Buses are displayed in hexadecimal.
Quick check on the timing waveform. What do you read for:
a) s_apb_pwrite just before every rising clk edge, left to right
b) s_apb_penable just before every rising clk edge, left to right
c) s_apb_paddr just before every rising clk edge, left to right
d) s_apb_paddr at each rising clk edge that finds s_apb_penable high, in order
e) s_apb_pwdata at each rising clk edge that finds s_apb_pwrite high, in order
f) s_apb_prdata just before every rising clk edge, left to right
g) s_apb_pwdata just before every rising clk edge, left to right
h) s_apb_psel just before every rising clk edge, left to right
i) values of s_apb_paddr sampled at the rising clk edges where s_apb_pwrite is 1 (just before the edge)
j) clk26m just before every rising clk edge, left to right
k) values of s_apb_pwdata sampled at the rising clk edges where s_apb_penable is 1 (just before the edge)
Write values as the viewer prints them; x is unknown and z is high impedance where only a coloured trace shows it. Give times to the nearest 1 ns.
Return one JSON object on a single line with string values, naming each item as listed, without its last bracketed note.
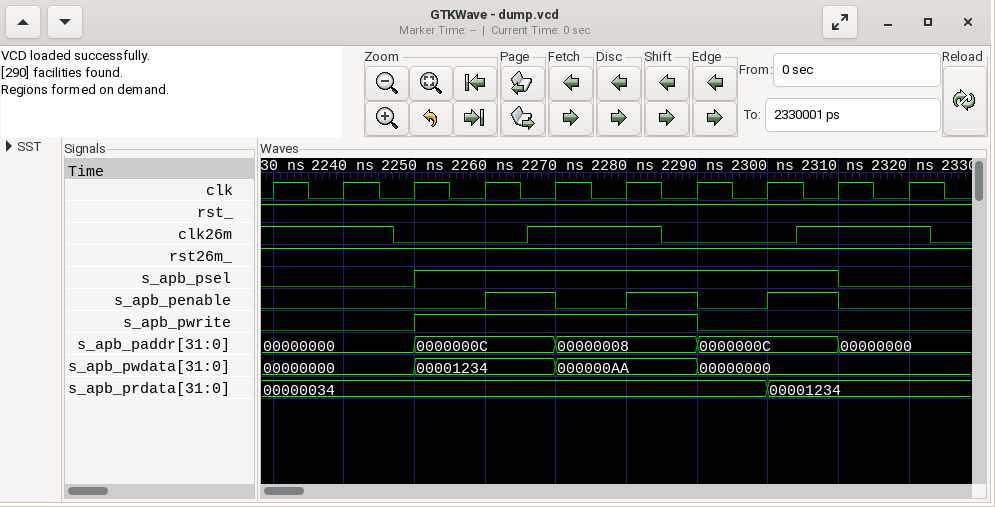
{"s_apb_pwrite just before every rising clk edge, left to right": "0 0 0 1 1 1 1 0 0 0", "s_apb_penable just before every rising clk edge, left to right": "0 0 0 0 1 0 1 0 1 0", "s_apb_paddr just before every rising clk edge, left to right": "00000000, 00000000, 00000000, 0000000C, 0000000C, 00000008, 00000008, 0000000C, 0000000C, 00000000", "s_apb_paddr at each rising clk edge that finds s_apb_penable high, in order": "0000000C, 00000008, 0000000C", "s_apb_pwdata at each rising clk edge that finds s_apb_pwrite high, in order": "00001234, 00001234, 000000AA, 000000AA", "s_apb_prdata just before every rising clk edge, left to right": "00000034, 00000034, 00000034, 00000034, 00000034, 00000034, 00000034, 00000034, 00001234, 00001234", "s_apb_pwdata just before every rising clk edge, left to right": "00000000, 00000000, 00000000, 00001234, 00001234, 000000AA, 000000AA, 00000000, 00000000, 00000000", "s_apb_psel just before every rising clk edge, left to right": "0 0 0 1 1 1 1 1 1 0", "values of s_apb_paddr sampled at the rising clk edges where s_apb_pwrite is 1": "0000000C, 0000000C, 00000008, 00000008", "clk26m just before every rising clk edge, left to right": "1 1 0 0 1 1 0 0 1 1", "values of s_apb_pwdata sampled at the rising clk edges where s_apb_penable is 1": "00001234, 000000AA, 00000000"}
